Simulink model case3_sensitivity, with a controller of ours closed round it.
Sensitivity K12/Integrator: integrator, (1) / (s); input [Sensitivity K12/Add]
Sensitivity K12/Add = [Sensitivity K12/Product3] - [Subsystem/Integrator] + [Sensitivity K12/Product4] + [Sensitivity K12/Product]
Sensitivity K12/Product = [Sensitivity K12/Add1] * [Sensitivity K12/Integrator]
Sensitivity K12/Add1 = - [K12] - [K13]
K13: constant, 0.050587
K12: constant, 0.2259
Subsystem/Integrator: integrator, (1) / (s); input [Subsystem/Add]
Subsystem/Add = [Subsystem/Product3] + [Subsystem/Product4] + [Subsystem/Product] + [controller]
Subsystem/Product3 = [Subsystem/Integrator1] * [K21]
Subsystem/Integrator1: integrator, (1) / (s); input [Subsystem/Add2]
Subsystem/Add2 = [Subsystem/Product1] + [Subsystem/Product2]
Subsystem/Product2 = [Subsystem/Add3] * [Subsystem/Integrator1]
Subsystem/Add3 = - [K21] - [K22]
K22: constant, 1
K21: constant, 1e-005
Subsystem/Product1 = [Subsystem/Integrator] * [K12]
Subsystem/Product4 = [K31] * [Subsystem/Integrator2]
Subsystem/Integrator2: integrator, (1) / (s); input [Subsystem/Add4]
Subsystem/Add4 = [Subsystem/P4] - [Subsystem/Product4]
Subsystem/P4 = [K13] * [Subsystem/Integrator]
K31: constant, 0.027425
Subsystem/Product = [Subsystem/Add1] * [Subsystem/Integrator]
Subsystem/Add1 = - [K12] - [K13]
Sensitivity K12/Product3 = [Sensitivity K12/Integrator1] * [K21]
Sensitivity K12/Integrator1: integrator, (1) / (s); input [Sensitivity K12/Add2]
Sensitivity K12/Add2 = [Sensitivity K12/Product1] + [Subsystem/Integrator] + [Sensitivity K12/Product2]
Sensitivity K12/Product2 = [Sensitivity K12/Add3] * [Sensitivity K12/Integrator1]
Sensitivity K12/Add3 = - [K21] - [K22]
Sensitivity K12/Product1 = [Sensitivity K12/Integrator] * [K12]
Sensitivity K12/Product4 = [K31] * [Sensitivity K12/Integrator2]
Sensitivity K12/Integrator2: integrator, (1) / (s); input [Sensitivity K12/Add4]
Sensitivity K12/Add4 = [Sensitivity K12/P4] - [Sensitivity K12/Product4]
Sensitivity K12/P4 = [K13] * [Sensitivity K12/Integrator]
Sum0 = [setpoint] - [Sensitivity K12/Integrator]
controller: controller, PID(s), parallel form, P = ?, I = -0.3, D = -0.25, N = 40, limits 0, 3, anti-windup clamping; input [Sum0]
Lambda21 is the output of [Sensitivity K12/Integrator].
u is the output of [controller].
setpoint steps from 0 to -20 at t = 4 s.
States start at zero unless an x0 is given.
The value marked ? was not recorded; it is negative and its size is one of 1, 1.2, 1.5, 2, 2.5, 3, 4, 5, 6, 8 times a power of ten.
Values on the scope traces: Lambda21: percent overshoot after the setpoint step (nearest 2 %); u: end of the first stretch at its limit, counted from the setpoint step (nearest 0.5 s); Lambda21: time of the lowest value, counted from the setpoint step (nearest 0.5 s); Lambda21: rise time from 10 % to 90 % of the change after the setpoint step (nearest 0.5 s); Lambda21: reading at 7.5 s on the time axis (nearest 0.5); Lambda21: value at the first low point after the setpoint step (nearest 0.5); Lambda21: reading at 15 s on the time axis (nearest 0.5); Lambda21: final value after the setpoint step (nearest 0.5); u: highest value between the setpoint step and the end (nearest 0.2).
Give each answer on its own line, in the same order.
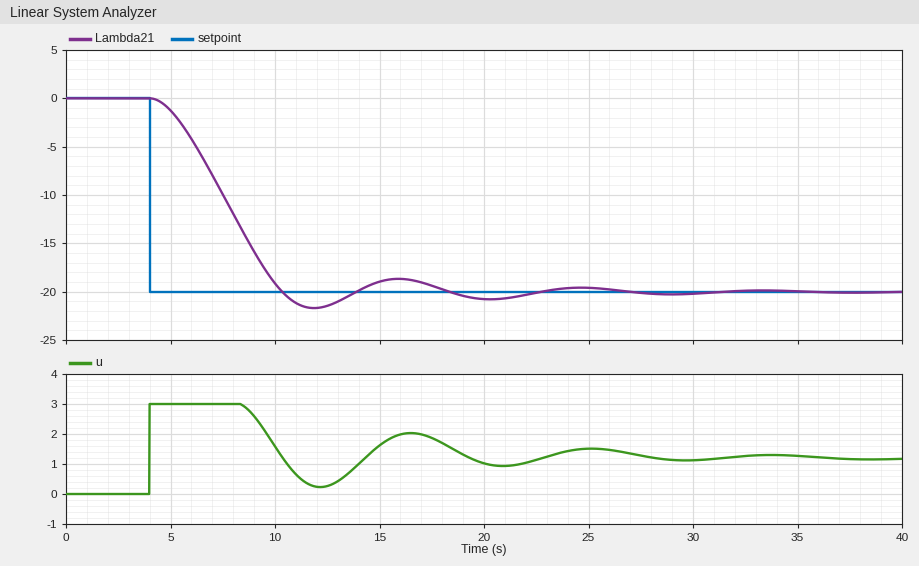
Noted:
8 %
4.5 s
8.0 s
4.5 s
-10.0
-21.5
-19.0
-20.0
3.0
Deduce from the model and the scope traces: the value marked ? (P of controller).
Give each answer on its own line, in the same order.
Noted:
-0.6
